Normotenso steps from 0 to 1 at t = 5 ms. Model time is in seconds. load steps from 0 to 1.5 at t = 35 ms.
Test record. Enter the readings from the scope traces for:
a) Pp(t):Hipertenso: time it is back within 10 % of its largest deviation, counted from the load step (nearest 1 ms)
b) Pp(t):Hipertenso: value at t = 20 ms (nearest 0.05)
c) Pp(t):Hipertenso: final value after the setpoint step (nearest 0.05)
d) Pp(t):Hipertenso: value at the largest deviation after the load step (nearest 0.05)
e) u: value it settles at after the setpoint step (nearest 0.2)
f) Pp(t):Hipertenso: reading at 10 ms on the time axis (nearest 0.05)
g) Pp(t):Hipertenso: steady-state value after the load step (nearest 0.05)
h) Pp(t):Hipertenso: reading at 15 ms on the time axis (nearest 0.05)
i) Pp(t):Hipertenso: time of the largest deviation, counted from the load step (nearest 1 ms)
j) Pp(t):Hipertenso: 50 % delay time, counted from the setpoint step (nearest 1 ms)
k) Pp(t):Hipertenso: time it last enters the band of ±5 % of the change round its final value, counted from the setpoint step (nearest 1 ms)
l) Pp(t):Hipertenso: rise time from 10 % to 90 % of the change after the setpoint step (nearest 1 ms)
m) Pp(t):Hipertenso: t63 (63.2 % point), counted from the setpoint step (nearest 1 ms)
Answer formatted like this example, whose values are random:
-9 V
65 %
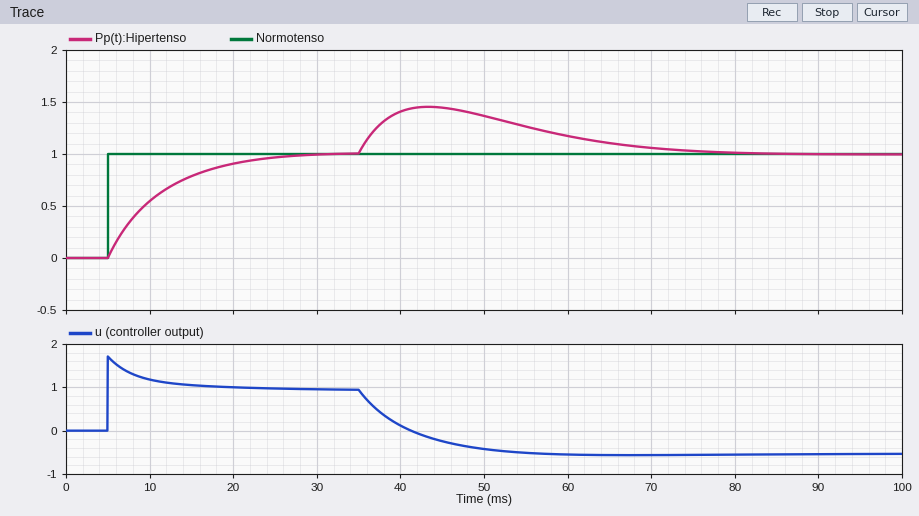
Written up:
37 ms
0.90
1.00
1.45
1.0
0.55
1.00
0.80
8 ms
4 ms
18 ms
14 ms
6 ms
